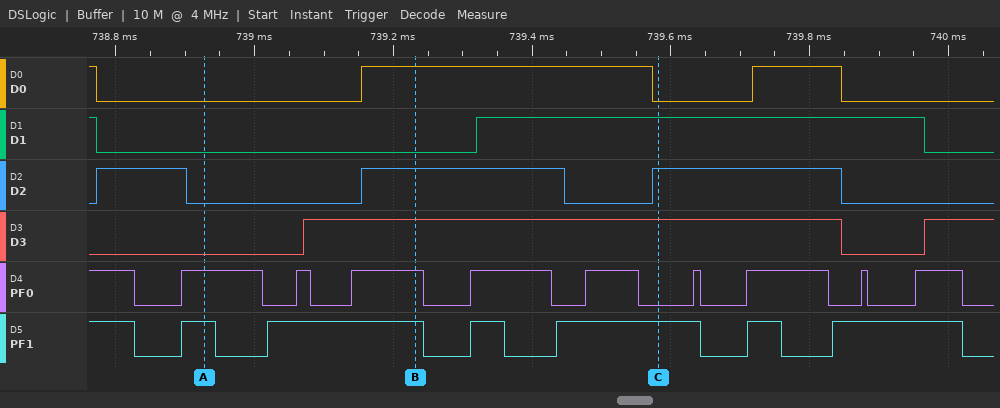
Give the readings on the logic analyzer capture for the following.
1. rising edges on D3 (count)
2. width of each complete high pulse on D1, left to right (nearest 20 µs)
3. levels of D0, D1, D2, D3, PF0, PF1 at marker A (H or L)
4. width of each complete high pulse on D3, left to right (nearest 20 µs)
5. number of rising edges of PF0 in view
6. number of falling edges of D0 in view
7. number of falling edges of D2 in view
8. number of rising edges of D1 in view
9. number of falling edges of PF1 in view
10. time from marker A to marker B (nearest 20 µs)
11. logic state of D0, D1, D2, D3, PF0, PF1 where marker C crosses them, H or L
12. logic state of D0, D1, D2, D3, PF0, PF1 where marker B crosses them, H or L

2
640 µs
D0=L, D1=L, D2=L, D3=L, PF0=H, PF1=H
780 µs
9
3
3
1
7
300 µs
D0=L, D1=H, D2=H, D3=H, PF0=L, PF1=H
D0=H, D1=L, D2=H, D3=H, PF0=H, PF1=H
